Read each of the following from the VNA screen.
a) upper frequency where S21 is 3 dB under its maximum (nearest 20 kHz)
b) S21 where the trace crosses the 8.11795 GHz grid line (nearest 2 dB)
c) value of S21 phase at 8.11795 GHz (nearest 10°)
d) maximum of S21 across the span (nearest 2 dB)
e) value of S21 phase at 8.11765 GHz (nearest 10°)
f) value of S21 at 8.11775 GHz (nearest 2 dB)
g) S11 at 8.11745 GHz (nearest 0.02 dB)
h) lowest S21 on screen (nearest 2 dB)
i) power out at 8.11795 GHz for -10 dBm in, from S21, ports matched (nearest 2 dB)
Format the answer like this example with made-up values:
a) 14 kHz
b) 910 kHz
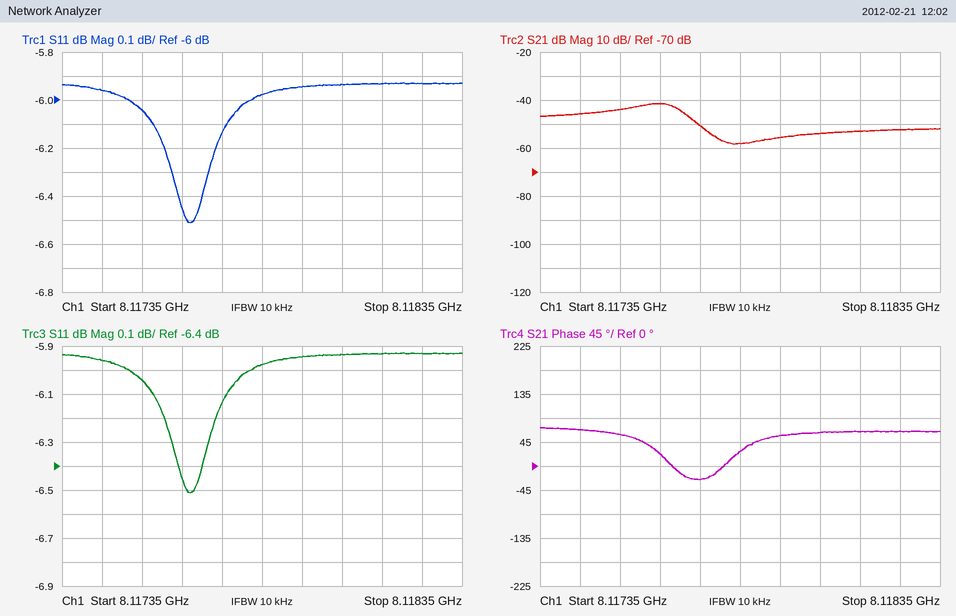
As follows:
a) 8.11770 GHz
b) -56 dB
c) 60°
d) -42 dB
e) 20°
f) -50 dB
g) -5.96 dB
h) -58 dB
i) -66 dBm
